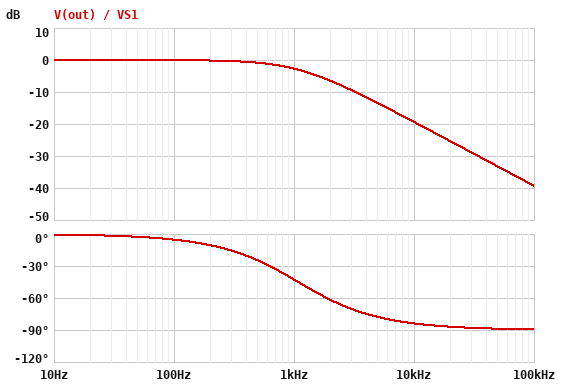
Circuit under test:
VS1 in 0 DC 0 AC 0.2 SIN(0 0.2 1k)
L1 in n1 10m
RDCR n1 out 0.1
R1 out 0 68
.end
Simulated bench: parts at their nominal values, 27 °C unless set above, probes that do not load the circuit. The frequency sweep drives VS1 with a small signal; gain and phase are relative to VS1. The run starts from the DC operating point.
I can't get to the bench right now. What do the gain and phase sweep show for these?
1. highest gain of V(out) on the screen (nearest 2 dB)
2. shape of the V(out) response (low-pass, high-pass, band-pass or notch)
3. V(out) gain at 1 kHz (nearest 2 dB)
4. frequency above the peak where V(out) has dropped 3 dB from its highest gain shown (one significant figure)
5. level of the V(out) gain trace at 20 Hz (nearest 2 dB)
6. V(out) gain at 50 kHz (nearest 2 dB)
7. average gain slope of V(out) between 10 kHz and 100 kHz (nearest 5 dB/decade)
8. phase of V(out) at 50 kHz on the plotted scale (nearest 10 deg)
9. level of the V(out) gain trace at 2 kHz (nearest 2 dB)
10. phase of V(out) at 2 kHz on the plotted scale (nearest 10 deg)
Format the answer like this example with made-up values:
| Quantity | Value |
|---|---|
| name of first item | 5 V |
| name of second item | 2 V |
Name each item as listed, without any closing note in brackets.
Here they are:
| Quantity | Value |
|---|---|
| highest gain of V(out) on the screen | 0 dB |
| shape of the V(out) response | low-pass |
| V(out) gain at 1 kHz | -2 dB |
| frequency above the peak where V(out) has dropped 3 dB from its highest gain shown | 1 kHz |
| level of the V(out) gain trace at 20 Hz | 0 dB |
| V(out) gain at 50 kHz | -34 dB |
| average gain slope of V(out) between 10 kHz and 100 kHz | -20 dB/decade |
| phase of V(out) at 50 kHz on the plotted scale | -90 deg |
| level of the V(out) gain trace at 2 kHz | -6 dB |
| phase of V(out) at 2 kHz on the plotted scale | -60 deg |
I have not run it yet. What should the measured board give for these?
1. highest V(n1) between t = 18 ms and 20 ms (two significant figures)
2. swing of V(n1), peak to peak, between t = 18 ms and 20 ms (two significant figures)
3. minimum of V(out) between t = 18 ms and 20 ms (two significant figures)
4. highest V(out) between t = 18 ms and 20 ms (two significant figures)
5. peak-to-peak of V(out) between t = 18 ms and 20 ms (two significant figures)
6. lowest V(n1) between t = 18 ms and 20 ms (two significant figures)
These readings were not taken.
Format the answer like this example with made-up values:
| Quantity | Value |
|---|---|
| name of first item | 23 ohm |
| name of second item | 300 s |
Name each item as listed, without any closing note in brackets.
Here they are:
| Quantity | Value |
|---|---|
| highest V(n1) between t = 18 ms and 20 ms | 150 mV |
| swing of V(n1), peak to peak, between t = 18 ms and 20 ms | 290 mV |
| minimum of V(out) between t = 18 ms and 20 ms | -150 mV |
| highest V(out) between t = 18 ms and 20 ms | 150 mV |
| peak-to-peak of V(out) between t = 18 ms and 20 ms | 290 mV |
| lowest V(n1) between t = 18 ms and 20 ms | -150 mV |
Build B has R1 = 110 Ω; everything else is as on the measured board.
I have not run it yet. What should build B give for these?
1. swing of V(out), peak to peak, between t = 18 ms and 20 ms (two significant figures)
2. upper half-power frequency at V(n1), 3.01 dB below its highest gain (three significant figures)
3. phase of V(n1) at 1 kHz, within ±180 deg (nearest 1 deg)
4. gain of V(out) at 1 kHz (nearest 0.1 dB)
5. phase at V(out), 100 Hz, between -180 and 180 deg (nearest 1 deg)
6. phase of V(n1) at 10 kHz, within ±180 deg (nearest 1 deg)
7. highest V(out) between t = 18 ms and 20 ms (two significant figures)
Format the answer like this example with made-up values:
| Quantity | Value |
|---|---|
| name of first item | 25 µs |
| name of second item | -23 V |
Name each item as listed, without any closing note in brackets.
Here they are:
| Quantity | Value |
|---|---|
| swing of V(out), peak to peak, between t = 18 ms and 20 ms | 350 mV |
| upper half-power frequency at V(n1), 3.01 dB below its highest gain | 1.75 kHz |
| phase of V(n1) at 1 kHz, within ±180 deg | -30 deg |
| gain of V(out) at 1 kHz | -1.2 dB |
| phase at V(out), 100 Hz, between -180 and 180 deg | -3 deg |
| phase of V(n1) at 10 kHz, within ±180 deg | -80 deg |
| highest V(out) between t = 18 ms and 20 ms | 170 mV |
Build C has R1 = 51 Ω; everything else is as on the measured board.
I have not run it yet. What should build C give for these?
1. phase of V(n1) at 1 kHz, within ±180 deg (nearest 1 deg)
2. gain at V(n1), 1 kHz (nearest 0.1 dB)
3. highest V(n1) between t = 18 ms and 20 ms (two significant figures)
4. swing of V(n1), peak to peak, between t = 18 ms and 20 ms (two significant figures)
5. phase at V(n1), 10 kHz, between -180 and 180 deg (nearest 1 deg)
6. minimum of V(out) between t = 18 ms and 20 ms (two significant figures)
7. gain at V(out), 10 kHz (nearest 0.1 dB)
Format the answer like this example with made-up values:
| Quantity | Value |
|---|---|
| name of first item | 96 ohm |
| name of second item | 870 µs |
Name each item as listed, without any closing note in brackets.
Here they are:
| Quantity | Value |
|---|---|
| phase of V(n1) at 1 kHz, within ±180 deg | -51 deg |
| gain at V(n1), 1 kHz | -4.0 dB |
| highest V(n1) between t = 18 ms and 20 ms | 130 mV |
| swing of V(n1), peak to peak, between t = 18 ms and 20 ms | 250 mV |
| phase at V(n1), 10 kHz, between -180 and 180 deg | -85 deg |
| minimum of V(out) between t = 18 ms and 20 ms | -130 mV |
| gain at V(out), 10 kHz | -21.8 dB |
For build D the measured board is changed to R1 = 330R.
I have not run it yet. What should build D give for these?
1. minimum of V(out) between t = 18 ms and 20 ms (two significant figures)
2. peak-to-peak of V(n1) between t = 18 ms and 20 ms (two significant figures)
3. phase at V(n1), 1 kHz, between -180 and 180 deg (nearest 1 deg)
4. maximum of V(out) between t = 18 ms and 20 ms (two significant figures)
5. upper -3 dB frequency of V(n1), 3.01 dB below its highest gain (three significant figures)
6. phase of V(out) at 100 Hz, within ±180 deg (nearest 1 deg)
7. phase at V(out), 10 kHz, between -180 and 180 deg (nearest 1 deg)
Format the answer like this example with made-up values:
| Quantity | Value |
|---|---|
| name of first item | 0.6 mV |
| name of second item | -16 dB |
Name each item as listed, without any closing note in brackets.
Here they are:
| Quantity | Value |
|---|---|
| minimum of V(out) between t = 18 ms and 20 ms | -200 mV |
| peak-to-peak of V(n1) between t = 18 ms and 20 ms | 390 mV |
| phase at V(n1), 1 kHz, between -180 and 180 deg | -11 deg |
| maximum of V(out) between t = 18 ms and 20 ms | 200 mV |
| upper -3 dB frequency of V(n1), 3.01 dB below its highest gain | 5.25 kHz |
| phase of V(out) at 100 Hz, within ±180 deg | -1 deg |
| phase at V(out), 10 kHz, between -180 and 180 deg | -62 deg |
